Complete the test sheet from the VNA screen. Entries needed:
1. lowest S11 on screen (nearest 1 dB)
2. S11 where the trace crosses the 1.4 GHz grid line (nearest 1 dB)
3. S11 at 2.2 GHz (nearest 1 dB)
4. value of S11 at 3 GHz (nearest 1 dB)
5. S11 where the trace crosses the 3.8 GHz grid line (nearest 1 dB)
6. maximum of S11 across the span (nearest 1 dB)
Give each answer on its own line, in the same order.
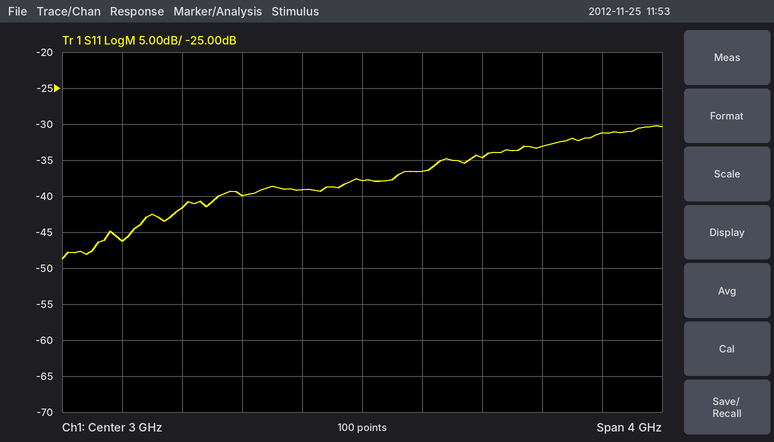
-49 dB
-46 dB
-40 dB
-38 dB
-35 dB
-30 dB
